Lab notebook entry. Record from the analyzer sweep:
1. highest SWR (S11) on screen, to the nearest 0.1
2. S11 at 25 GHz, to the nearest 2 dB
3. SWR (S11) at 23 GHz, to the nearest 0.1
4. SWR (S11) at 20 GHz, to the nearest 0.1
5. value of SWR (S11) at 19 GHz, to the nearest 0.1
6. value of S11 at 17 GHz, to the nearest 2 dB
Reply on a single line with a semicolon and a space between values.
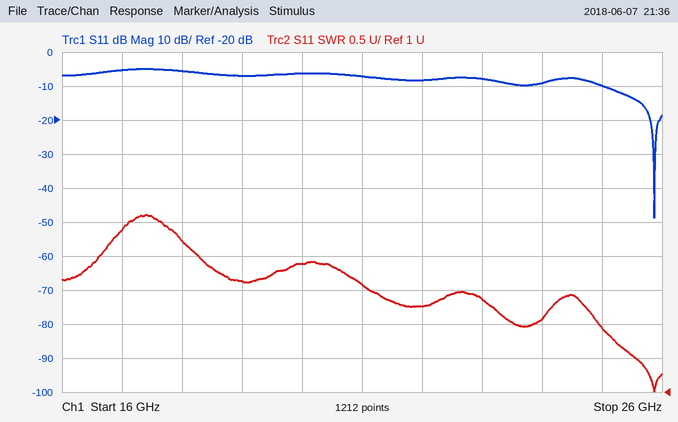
3.6; -10 dB; 2.4; 2.9; 2.6; -6 dB
